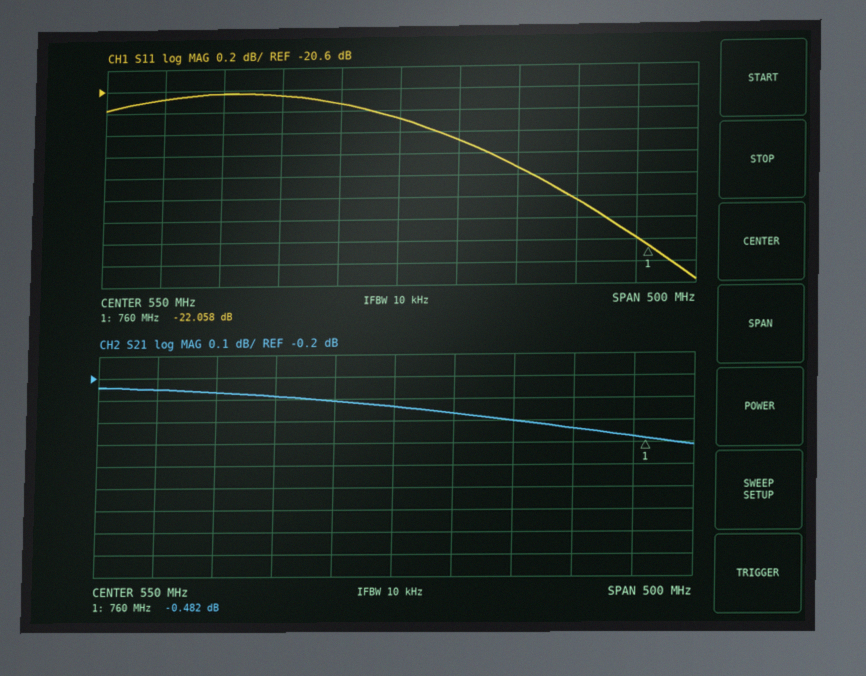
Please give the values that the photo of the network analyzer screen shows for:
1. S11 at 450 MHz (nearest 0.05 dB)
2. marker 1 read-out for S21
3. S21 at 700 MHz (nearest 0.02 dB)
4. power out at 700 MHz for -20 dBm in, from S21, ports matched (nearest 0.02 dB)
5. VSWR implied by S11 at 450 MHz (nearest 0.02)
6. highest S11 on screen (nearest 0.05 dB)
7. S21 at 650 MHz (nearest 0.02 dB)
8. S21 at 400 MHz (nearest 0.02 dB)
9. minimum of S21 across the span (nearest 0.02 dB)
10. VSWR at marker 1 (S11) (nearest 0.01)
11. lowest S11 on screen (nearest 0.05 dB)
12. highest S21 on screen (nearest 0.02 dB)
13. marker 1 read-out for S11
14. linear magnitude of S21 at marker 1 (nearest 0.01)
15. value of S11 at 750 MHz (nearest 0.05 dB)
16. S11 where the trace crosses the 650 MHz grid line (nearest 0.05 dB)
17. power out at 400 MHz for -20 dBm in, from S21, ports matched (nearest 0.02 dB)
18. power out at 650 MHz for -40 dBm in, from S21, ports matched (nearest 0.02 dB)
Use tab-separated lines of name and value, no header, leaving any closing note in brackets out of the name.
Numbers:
S11 at 450 MHz	-20.65 dB
marker 1 read-out for S21	-0.482 dB
S21 at 700 MHz	-0.44 dB
power out at 700 MHz for -20 dBm in, from S21, ports matched	-20.44 dBm
VSWR implied by S11 at 450 MHz	1.20
highest S11 on screen	-20.65 dB
S21 at 650 MHz	-0.40 dB
S21 at 400 MHz	-0.26 dB
minimum of S21 across the span	-0.52 dB
VSWR at marker 1 (S11)	1.17
lowest S11 on screen	-22.35 dB
highest S21 on screen	-0.24 dB
marker 1 read-out for S11	-22.058 dB
linear magnitude of S21 at marker 1	0.95
value of S11 at 750 MHz	-22.00 dB
S11 where the trace crosses the 650 MHz grid line	-21.35 dB
power out at 400 MHz for -20 dBm in, from S21, ports matched	-20.26 dBm
power out at 650 MHz for -40 dBm in, from S21, ports matched	-40.40 dBm
